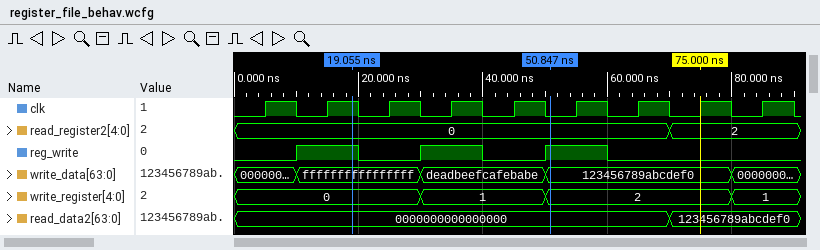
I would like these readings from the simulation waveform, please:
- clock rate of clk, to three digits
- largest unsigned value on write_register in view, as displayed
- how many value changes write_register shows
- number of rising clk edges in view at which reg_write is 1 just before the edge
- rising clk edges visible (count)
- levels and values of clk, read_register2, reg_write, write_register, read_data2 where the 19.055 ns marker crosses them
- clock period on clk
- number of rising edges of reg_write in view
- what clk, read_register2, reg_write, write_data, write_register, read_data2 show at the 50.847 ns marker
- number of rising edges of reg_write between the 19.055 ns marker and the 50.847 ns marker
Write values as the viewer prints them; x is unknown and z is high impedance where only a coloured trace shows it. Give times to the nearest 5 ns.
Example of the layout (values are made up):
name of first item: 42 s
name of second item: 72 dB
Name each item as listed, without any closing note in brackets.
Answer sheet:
clock rate of clk, to three digits: 100 MHz
largest unsigned value on write_register in view, as displayed: 2
how many value changes write_register shows: 3
number of rising clk edges in view at which reg_write is 1 just before the edge: 3
rising clk edges visible: 9
levels and values of clk, read_register2, reg_write, write_register, read_data2 where the 19.055 ns marker crosses them: clk=1, read_register2=0, reg_write=1, write_register=0, read_data2=0000000000000000
clock period on clk: 10 ns
number of rising edges of reg_write in view: 3
what clk, read_register2, reg_write, write_data, write_register, read_data2 show at the 50.847 ns marker: clk=0, read_register2=0, reg_write=1, write_data=123456789abcdef0, write_register=2, read_data2=0000000000000000
number of rising edges of reg_write between the 19.055 ns marker and the 50.847 ns marker: 2
